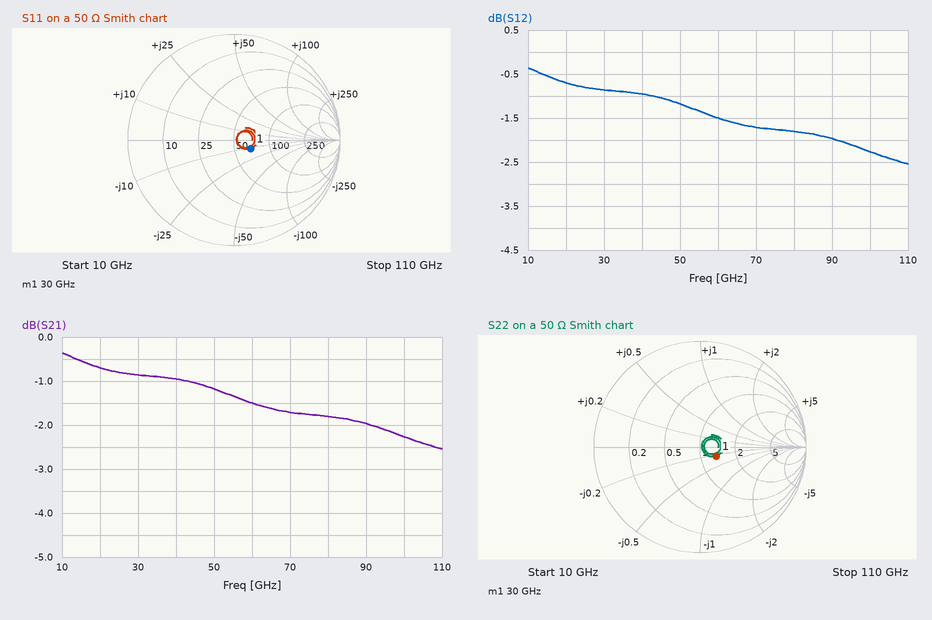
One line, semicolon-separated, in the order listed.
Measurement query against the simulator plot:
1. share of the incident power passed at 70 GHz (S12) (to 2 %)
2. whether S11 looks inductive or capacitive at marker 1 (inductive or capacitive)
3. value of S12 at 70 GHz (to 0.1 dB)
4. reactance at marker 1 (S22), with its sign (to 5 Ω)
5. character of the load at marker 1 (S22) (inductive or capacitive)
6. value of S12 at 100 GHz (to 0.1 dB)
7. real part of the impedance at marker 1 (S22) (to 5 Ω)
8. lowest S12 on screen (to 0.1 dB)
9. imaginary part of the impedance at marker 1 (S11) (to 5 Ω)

68 %; capacitive; -1.7 dB; -10 Ω; capacitive; -2.3 dB; 65 Ω; -2.5 dB; -10 Ω
